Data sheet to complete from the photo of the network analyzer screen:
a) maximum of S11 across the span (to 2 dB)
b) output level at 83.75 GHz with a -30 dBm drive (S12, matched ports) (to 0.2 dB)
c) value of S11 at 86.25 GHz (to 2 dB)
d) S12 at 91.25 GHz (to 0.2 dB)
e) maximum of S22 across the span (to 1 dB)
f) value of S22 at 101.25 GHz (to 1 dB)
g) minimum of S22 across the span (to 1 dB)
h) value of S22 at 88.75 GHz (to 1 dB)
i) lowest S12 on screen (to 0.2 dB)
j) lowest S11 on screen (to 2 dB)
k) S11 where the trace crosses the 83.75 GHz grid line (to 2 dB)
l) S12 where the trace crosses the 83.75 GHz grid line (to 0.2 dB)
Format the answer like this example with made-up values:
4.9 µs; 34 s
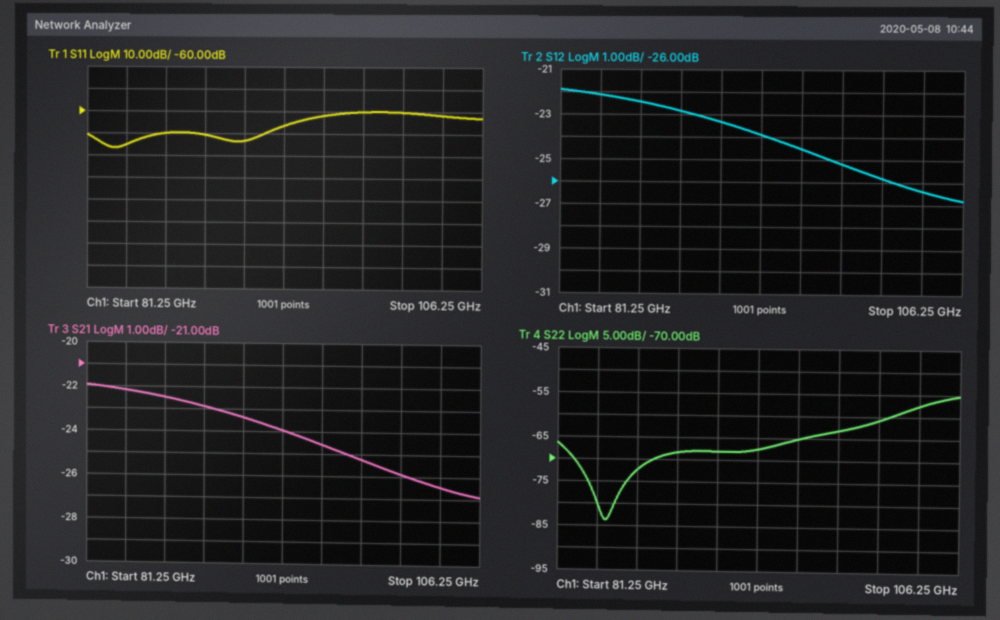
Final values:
-60 dB; -52.2 dBm; -70 dB; -23.4 dB; -55 dB; -61 dB; -84 dB; -68 dB; -26.8 dB; -76 dB; -76 dB; -22.2 dB
